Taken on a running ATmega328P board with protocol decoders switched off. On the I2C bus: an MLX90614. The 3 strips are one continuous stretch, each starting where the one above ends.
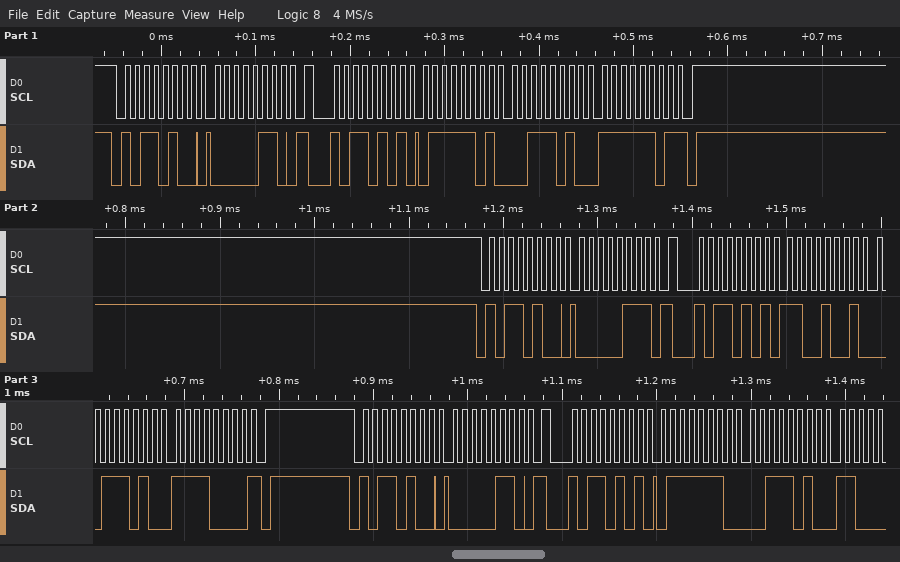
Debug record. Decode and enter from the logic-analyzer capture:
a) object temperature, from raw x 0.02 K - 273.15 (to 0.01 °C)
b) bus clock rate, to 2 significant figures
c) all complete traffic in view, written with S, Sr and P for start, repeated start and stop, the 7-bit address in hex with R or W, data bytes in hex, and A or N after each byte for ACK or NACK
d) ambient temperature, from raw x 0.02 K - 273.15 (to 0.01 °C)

27.83 °C
100 kHz
S 5AW A 06 A Sr 5AR A 7D A 3A A FD N P S 5AW A 07 A Sr 5AR A C9 A 3A A F0 N P S 5AW A 06 A Sr 5AR A 7E A 3A A
26.31 °C
